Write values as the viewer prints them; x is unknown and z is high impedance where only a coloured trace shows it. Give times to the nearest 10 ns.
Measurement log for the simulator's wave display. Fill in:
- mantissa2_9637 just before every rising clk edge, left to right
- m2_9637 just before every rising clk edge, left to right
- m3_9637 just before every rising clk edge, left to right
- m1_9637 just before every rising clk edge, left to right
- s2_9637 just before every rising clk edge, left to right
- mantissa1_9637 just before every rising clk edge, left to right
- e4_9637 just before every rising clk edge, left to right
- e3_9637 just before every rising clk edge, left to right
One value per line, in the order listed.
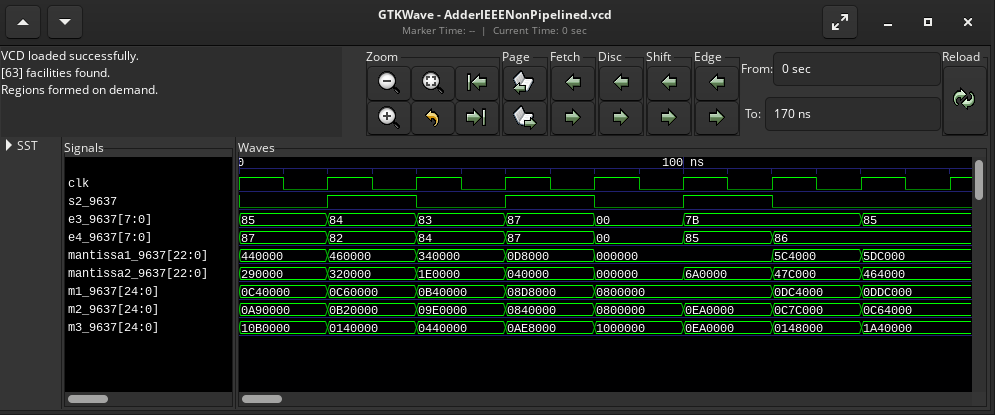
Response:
290000, 320000, 1E0000, 040000, 000000, 6A0000, 47C000, 464000
0A90000, 0B20000, 09E0000, 0840000, 0800000, 0EA0000, 0C7C000, 0C64000
10B0000, 0140000, 0440000, 0AE8000, 1000000, 0EA0000, 0148000, 1A40000
0C40000, 0C60000, 0B40000, 08D8000, 0800000, 0800000, 0DC4000, 0DDC000
0 1 0 1 0 1 0 0
440000, 460000, 340000, 0D8000, 000000, 000000, 5C4000, 5DC000
87, 82, 84, 87, 00, 85, 86, 86
85, 84, 83, 87, 00, 7B, 7B, 85
